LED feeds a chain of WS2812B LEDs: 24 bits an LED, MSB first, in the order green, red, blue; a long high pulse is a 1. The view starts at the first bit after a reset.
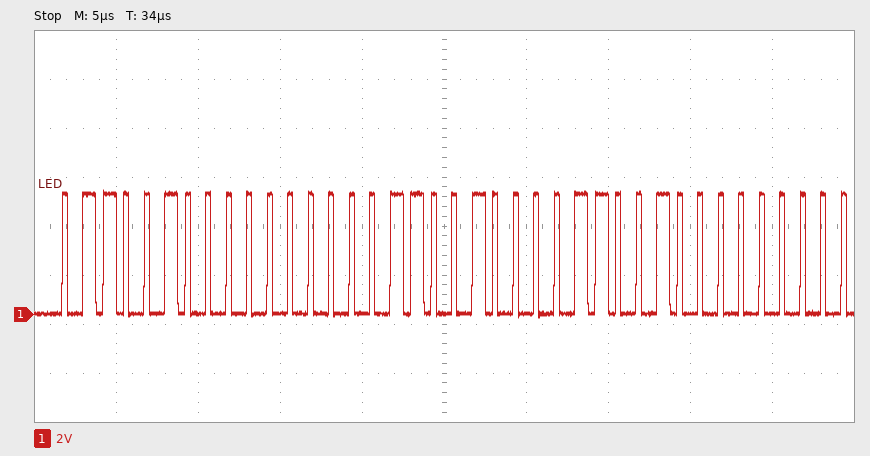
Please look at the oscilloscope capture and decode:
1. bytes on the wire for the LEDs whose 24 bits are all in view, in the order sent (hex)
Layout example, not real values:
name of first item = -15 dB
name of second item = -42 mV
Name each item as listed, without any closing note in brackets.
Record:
bytes on the wire for the LEDs whose 24 bits are all in view, in the order sent = 64 00 C8
